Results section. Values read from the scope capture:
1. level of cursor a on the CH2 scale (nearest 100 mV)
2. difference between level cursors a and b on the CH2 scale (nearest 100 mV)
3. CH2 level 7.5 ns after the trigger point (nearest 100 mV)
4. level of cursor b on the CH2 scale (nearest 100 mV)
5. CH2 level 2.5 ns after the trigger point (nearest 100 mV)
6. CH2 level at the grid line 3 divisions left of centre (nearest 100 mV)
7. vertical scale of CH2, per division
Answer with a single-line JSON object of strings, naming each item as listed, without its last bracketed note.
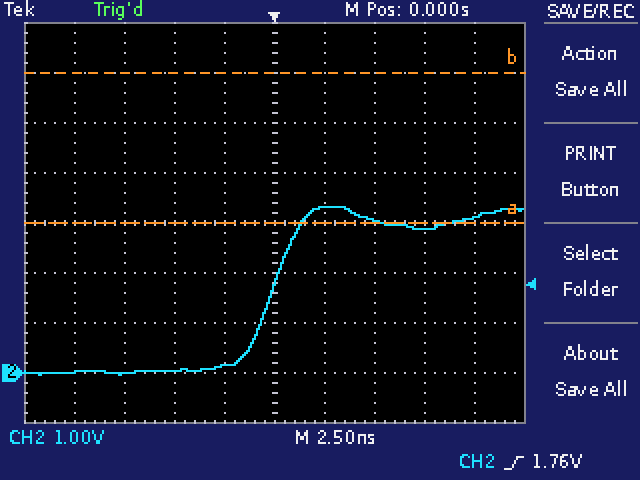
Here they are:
{"level of cursor a on the CH2 scale": "3.0 V", "difference between level cursors a and b on the CH2 scale": "3.0 V", "CH2 level 7.5 ns after the trigger point": "2.9 V", "level of cursor b on the CH2 scale": "6.0 V", "CH2 level 2.5 ns after the trigger point": "3.3 V", "CH2 level at the grid line 3 divisions left of centre": "0.0 V", "vertical scale of CH2, per division": "1 V"}
